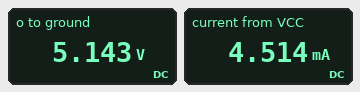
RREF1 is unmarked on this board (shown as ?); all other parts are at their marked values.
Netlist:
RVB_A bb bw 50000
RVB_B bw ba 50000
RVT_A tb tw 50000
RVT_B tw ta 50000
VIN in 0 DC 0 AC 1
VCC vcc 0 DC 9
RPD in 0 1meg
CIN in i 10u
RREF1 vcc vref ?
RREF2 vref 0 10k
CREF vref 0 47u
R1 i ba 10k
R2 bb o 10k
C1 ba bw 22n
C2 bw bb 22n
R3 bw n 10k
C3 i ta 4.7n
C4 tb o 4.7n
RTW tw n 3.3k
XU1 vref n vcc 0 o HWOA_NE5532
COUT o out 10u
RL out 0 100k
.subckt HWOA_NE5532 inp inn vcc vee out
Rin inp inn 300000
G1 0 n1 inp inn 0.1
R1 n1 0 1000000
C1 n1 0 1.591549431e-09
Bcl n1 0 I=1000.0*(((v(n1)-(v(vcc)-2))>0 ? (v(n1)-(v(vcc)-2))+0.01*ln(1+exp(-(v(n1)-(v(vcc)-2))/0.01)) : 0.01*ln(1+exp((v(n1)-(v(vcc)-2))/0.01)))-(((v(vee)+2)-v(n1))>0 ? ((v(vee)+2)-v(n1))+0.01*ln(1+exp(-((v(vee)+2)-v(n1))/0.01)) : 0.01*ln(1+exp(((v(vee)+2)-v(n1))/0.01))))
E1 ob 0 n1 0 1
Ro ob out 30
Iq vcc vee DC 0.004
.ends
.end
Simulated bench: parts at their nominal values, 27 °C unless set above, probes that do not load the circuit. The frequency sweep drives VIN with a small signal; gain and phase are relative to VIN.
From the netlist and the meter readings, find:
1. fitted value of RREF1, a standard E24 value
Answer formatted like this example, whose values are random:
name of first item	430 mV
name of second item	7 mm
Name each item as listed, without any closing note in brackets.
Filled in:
fitted value of RREF1, a standard E24 value	7.5 kΩ
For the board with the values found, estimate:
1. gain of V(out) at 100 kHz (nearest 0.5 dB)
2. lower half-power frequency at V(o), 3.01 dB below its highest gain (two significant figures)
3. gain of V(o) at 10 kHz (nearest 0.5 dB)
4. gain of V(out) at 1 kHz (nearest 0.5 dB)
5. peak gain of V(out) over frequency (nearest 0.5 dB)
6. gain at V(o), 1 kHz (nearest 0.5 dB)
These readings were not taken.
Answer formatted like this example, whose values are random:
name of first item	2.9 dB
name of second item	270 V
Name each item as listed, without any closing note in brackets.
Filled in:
gain of V(out) at 100 kHz	0 dB
lower half-power frequency at V(o), 3.01 dB below its highest gain	270 mHz
gain of V(o) at 10 kHz	0 dB
gain of V(out) at 1 kHz	0 dB
peak gain of V(out) over frequency	0 dB
gain at V(o), 1 kHz	0 dB
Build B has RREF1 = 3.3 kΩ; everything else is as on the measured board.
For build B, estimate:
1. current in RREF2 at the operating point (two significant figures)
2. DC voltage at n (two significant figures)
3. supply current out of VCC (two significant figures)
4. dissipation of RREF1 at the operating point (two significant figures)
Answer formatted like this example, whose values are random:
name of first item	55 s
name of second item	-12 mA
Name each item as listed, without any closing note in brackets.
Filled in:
current in RREF2 at the operating point	680 µA
DC voltage at n	6.8 V
supply current out of VCC	4.7 mA
dissipation of RREF1 at the operating point	1.5 mW
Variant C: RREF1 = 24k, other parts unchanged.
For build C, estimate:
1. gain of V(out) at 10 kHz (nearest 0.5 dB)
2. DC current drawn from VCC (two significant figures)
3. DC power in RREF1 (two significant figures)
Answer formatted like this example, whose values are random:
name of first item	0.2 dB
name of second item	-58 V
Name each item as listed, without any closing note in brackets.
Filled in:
gain of V(out) at 10 kHz	0 dB
DC current drawn from VCC	4.3 mA
DC power in RREF1	1.7 mW
